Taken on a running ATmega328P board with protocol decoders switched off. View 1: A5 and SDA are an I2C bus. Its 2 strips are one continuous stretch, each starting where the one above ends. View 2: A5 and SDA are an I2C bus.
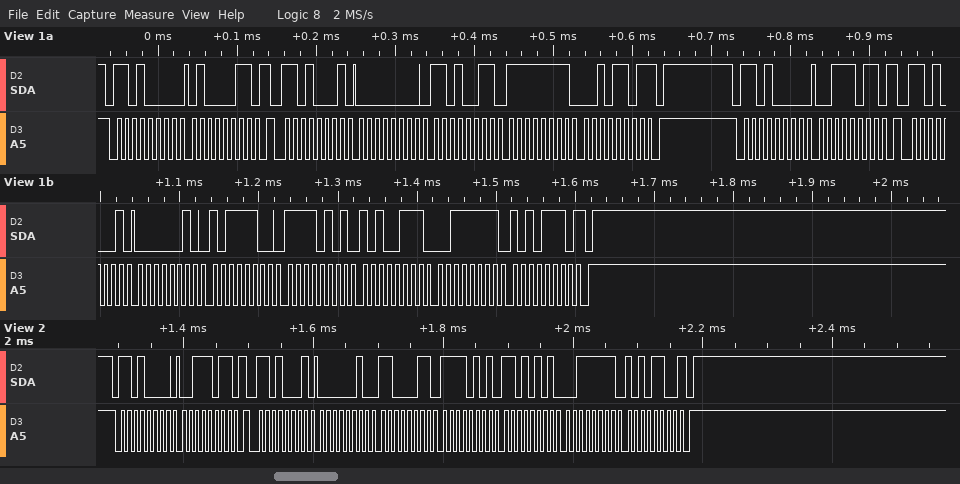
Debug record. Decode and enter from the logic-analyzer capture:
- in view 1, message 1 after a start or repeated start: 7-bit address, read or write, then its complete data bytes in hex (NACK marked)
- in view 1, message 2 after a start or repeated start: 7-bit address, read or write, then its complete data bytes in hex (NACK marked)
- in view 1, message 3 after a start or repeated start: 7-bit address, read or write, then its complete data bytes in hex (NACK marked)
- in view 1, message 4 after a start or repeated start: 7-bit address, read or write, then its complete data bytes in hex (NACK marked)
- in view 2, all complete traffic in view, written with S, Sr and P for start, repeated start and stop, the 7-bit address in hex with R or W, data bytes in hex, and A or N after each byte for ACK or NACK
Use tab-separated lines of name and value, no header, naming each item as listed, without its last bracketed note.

in view 1, message 1 after a start or repeated start: 7-bit address, read or write, then its complete data bytes in hex	0x68 write: 43
in view 1, message 2 after a start or repeated start: 7-bit address, read or write, then its complete data bytes in hex	0x68 read: 00 D3 FF 2D NACK
in view 1, message 3 after a start or repeated start: 7-bit address, read or write, then its complete data bytes in hex	0x68 write: 3B
in view 1, message 4 after a start or repeated start: 7-bit address, read or write, then its complete data bytes in hex	0x68 read: 02 BC F5 A7 3F AE NACK
in view 2, all complete traffic in view, written with S, Sr and P for start, repeated start and stop, the 7-bit address in hex with R or W, data bytes in hex, and A or N after each byte for ACK or NACK	S 68W A 3B A Sr 68R A 02 A C3 A F5 A D5 A 3F A AC N P
